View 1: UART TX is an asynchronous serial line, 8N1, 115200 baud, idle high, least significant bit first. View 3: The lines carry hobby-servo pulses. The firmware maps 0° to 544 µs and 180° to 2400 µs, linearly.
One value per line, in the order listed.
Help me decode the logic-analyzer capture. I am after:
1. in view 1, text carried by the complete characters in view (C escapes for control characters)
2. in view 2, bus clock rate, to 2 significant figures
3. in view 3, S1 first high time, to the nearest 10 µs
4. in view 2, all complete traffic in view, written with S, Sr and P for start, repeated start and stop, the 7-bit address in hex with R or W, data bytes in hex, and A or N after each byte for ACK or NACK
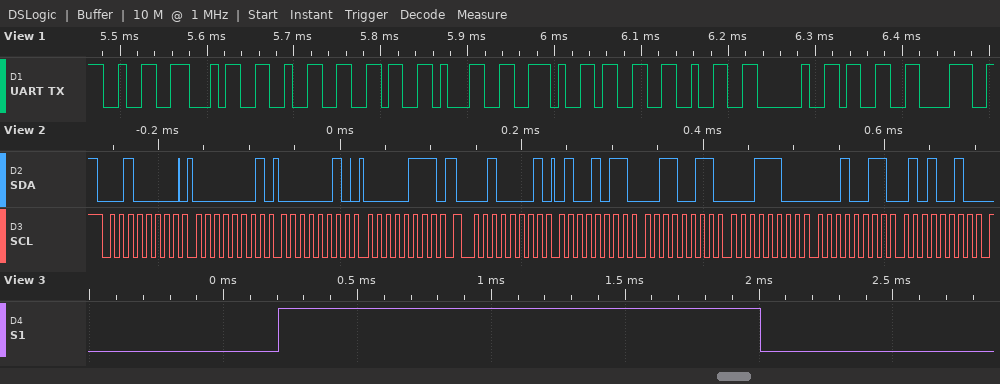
"24261.32 38"
100 kHz
1800 µs
S 10W A 01 A 02 A 07 A Sr 10R A 4B A 33 A 1C A 13 A 52 A
